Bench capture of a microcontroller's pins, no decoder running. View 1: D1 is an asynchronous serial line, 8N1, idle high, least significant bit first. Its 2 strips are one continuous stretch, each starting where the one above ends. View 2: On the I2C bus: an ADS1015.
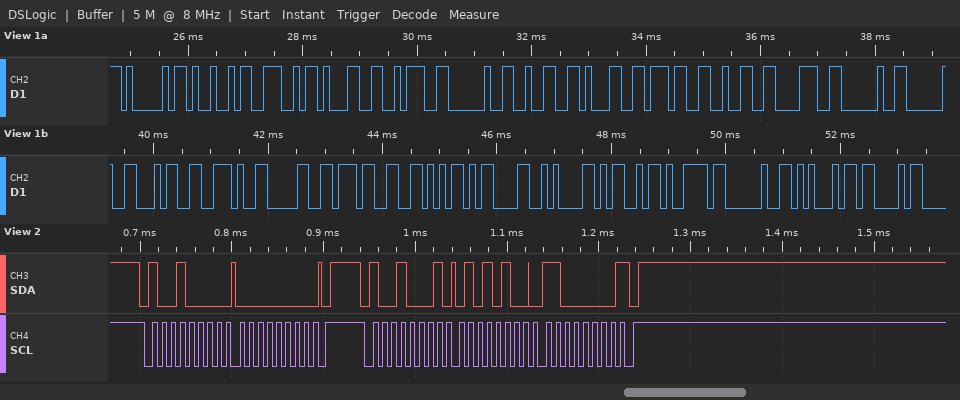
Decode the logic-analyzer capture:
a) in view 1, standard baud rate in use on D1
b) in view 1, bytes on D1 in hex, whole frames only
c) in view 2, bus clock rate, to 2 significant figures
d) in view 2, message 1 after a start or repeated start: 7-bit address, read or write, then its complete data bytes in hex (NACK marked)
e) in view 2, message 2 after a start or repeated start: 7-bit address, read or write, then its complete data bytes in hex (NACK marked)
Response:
9600 baud
41 49 4E 31 3A 20 32 31 37 32 38 20 20 34 2E 30 37 56 0D 0A 4D 79 20 45 43
100 kHz
0x48 write: 00
0x48 read: 54 C0 NACK
